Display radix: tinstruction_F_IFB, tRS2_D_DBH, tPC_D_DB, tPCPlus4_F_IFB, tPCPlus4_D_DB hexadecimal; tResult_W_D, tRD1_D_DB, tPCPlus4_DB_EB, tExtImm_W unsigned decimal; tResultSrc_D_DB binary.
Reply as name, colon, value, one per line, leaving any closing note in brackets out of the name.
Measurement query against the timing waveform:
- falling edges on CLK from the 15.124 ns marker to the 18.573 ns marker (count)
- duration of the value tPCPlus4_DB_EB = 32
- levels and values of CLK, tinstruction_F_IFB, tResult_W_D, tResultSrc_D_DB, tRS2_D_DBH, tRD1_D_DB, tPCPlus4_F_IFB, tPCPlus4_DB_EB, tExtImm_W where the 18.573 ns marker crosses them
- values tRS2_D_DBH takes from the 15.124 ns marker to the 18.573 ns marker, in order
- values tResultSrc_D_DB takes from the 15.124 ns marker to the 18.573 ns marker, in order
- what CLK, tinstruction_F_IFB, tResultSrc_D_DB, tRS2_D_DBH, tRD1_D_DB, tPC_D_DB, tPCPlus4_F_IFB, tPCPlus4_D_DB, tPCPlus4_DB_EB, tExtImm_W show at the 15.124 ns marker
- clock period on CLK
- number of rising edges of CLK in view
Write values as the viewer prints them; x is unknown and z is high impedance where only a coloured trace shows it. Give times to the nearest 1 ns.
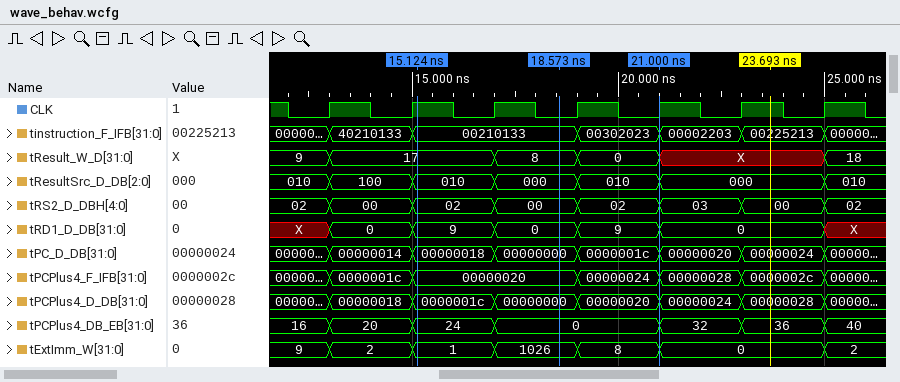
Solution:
falling edges on CLK from the 15.124 ns marker to the 18.573 ns marker: 2
duration of the value tPCPlus4_DB_EB = 32: 2 ns
levels and values of CLK, tinstruction_F_IFB, tResult_W_D, tResultSrc_D_DB, tRS2_D_DBH, tRD1_D_DB, tPCPlus4_F_IFB, tPCPlus4_DB_EB, tExtImm_W where the 18.573 ns marker crosses them: CLK=0, tinstruction_F_IFB=00210133, tResult_W_D=8, tResultSrc_D_DB=000, tRS2_D_DBH=00, tRD1_D_DB=0, tPCPlus4_F_IFB=00000020, tPCPlus4_DB_EB=0, tExtImm_W=1026
values tRS2_D_DBH takes from the 15.124 ns marker to the 18.573 ns marker, in order: 02, 00
values tResultSrc_D_DB takes from the 15.124 ns marker to the 18.573 ns marker, in order: 010, 000
what CLK, tinstruction_F_IFB, tResultSrc_D_DB, tRS2_D_DBH, tRD1_D_DB, tPC_D_DB, tPCPlus4_F_IFB, tPCPlus4_D_DB, tPCPlus4_DB_EB, tExtImm_W show at the 15.124 ns marker: CLK=1, tinstruction_F_IFB=00210133, tResultSrc_D_DB=010, tRS2_D_DBH=02, tRD1_D_DB=9, tPC_D_DB=00000018, tPCPlus4_F_IFB=00000020, tPCPlus4_D_DB=0000001c, tPCPlus4_DB_EB=24, tExtImm_W=1
clock period on CLK: 2 ns
number of rising edges of CLK in view: 7
